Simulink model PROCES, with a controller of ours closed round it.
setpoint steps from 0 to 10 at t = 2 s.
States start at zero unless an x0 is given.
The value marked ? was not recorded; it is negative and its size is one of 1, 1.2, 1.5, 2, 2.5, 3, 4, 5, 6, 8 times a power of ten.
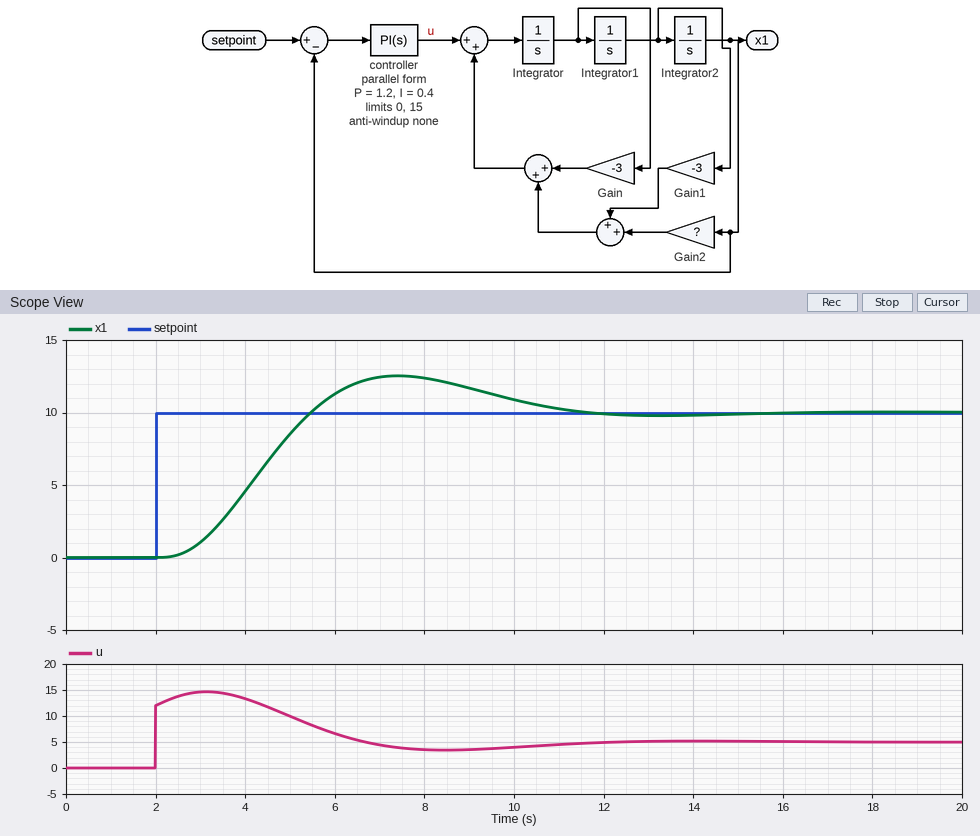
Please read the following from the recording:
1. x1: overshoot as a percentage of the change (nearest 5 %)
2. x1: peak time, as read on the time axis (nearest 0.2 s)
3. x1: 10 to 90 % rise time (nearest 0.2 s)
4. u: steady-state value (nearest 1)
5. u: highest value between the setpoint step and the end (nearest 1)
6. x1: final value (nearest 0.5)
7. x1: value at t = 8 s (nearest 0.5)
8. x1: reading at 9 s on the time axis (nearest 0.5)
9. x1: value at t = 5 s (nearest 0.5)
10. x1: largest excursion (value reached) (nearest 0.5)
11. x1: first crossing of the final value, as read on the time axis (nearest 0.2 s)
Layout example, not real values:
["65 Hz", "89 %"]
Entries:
["25 %", "7.4 s", "2.2 s", "5", "15", "10.0", "12.5", "11.5", "8.5", "12.5", "5.4 s"]
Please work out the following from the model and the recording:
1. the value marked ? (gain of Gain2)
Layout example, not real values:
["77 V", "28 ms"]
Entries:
["-0.5"]
